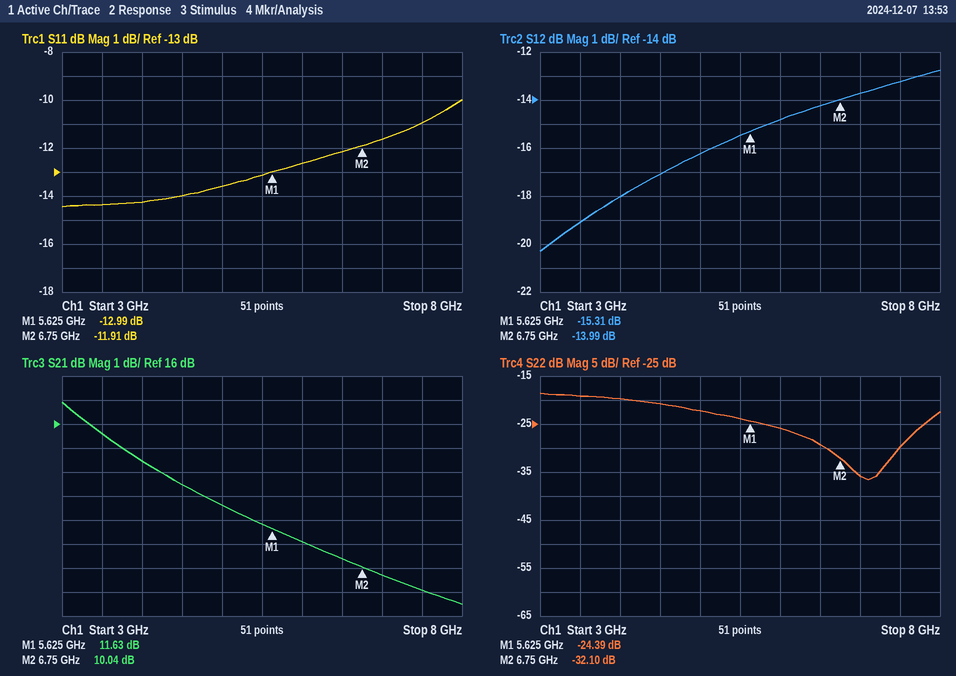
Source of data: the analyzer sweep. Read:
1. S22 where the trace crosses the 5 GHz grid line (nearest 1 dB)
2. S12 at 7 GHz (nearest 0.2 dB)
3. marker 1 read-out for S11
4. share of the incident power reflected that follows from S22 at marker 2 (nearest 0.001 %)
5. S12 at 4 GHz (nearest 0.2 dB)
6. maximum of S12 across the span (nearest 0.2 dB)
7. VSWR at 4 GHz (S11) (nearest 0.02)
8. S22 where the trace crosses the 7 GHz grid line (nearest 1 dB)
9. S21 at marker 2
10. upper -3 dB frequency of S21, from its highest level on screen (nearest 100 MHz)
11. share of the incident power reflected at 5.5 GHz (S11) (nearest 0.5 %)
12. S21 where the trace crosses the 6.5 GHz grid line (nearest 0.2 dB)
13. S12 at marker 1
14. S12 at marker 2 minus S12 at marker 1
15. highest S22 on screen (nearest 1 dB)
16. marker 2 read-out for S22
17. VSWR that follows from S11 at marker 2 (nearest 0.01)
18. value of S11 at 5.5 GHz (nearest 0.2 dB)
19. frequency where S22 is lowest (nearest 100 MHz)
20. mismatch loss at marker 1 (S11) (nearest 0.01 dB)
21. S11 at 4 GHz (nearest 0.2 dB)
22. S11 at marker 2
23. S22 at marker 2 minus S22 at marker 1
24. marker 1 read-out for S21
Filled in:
-22 dB
-13.8 dB
-12.99 dB
0.062 %
-18.0 dB
-12.8 dB
1.48
-36 dB
10.04 dB
4.3 GHz
5.0 %
10.4 dB
-15.31 dB
1.32 dB
-19 dB
-32.10 dB
1.68
-13.2 dB
7.1 GHz
0.22 dB
-14.2 dB
-11.91 dB
-7.71 dB
11.63 dB
